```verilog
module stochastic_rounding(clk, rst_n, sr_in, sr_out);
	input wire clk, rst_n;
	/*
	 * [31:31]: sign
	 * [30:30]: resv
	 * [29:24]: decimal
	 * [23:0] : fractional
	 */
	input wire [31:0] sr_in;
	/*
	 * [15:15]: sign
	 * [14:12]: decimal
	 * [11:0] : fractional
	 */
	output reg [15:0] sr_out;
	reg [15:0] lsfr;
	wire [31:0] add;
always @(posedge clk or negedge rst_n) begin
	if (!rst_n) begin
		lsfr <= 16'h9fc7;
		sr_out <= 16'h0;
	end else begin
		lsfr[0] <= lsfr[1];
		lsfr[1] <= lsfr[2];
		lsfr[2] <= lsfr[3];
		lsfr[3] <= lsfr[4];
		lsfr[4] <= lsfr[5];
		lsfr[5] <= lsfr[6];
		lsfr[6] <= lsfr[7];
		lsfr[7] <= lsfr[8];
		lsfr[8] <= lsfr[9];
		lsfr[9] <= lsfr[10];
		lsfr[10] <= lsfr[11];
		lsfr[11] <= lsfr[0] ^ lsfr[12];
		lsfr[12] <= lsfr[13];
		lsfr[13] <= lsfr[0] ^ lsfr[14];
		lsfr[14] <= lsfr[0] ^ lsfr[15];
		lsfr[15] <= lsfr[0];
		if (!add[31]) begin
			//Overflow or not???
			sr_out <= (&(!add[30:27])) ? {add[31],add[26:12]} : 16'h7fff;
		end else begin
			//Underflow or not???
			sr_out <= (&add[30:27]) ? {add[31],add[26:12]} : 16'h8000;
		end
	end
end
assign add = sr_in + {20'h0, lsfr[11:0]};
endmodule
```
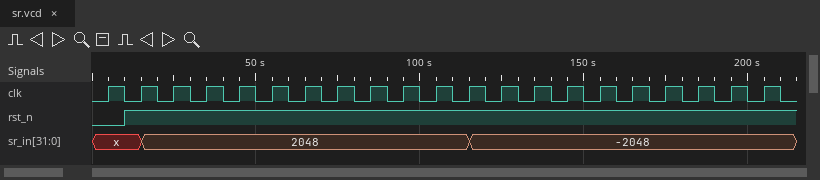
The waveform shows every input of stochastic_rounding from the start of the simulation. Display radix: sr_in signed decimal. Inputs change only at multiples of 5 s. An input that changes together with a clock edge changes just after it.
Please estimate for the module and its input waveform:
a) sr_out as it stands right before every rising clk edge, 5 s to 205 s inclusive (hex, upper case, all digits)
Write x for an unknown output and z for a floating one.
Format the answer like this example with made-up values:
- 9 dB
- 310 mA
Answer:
- 0000, 0000, x, 0000, 0001, 0000, 0001, 0001, 0000, 0000, 0001, 0000, 0001, FFFF, FFFF, 0000, FFFF, FFFF, 0000, FFFF, FFFF
